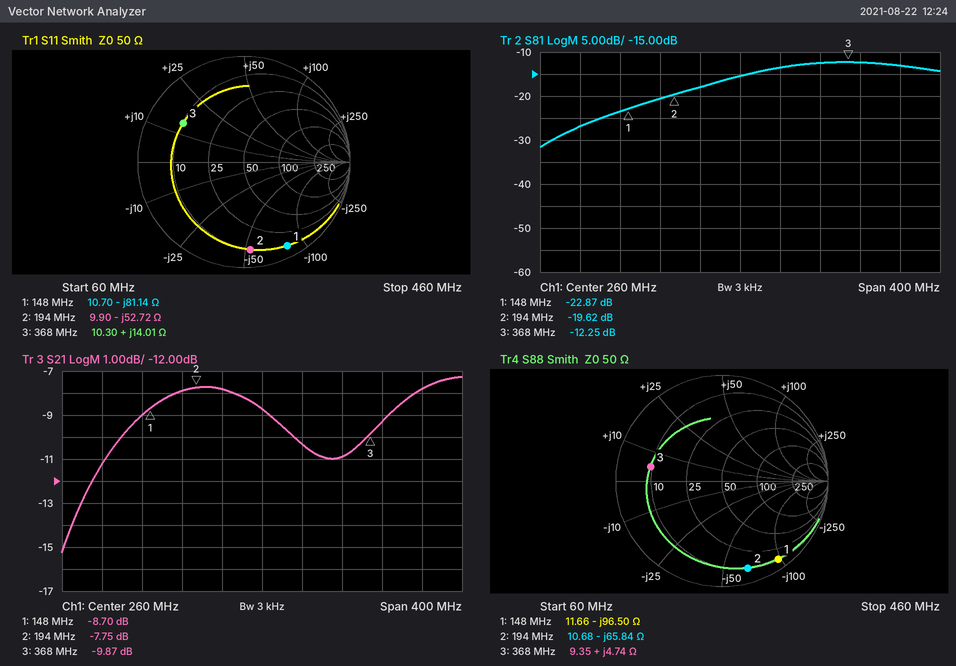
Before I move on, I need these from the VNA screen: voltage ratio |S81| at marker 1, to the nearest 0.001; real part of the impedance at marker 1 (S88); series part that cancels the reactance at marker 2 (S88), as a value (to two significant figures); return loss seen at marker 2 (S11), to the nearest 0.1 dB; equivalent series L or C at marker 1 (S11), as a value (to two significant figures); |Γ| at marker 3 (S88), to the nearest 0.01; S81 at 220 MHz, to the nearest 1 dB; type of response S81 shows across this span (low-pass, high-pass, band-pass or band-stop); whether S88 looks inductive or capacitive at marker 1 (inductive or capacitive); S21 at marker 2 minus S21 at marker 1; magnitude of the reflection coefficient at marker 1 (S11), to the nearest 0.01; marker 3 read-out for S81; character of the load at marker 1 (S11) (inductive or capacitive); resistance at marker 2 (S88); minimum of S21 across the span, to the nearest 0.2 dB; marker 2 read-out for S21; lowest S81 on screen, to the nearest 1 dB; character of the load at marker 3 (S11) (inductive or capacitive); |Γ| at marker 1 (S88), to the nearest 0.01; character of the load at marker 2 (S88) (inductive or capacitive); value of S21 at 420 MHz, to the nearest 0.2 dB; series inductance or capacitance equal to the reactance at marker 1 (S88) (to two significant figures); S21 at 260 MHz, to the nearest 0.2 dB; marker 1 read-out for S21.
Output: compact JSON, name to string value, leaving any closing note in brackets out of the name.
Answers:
{"voltage ratio |S81| at marker 1, to the nearest 0.001": "0.072", "real part of the impedance at marker 1": "11.66 Ω", "series part that cancels the reactance at marker 2 (S88), as a value": "54 nH", "return loss seen at marker 2 (S11), to the nearest 0.1 dB": "1.6 dB", "equivalent series L or C at marker 1 (S11), as a value": "13 pF", "|Γ| at marker 3 (S88), to the nearest 0.01": "0.69", "S81 at 220 MHz, to the nearest 1 dB": "-18 dB", "type of response S81 shows across this span": "high-pass", "whether S88 looks inductive or capacitive at marker 1": "capacitive", "S21 at marker 2 minus S21 at marker 1": "0.95 dB", "magnitude of the reflection coefficient at marker 1 (S11), to the nearest 0.01": "0.89", "marker 3 read-out for S81": "-12.25 dB", "character of the load at marker 1 (S11)": "capacitive", "resistance at marker 2": "10.68 Ω", "minimum of S21 across the span, to the nearest 0.2 dB": "-15.2 dB", "marker 2 read-out for S21": "-7.75 dB", "lowest S81 on screen, to the nearest 1 dB": "-32 dB", "character of the load at marker 3 (S11)": "inductive", "|Γ| at marker 1 (S88), to the nearest 0.01": "0.91", "character of the load at marker 2 (S88)": "capacitive", "value of S21 at 420 MHz, to the nearest 0.2 dB": "-7.8 dB", "series inductance or capacitance equal to the reactance at marker 1 (S88)": "11 pF", "S21 at 260 MHz, to the nearest 0.2 dB": "-8.8 dB", "marker 1 read-out for S21": "-8.70 dB"}
